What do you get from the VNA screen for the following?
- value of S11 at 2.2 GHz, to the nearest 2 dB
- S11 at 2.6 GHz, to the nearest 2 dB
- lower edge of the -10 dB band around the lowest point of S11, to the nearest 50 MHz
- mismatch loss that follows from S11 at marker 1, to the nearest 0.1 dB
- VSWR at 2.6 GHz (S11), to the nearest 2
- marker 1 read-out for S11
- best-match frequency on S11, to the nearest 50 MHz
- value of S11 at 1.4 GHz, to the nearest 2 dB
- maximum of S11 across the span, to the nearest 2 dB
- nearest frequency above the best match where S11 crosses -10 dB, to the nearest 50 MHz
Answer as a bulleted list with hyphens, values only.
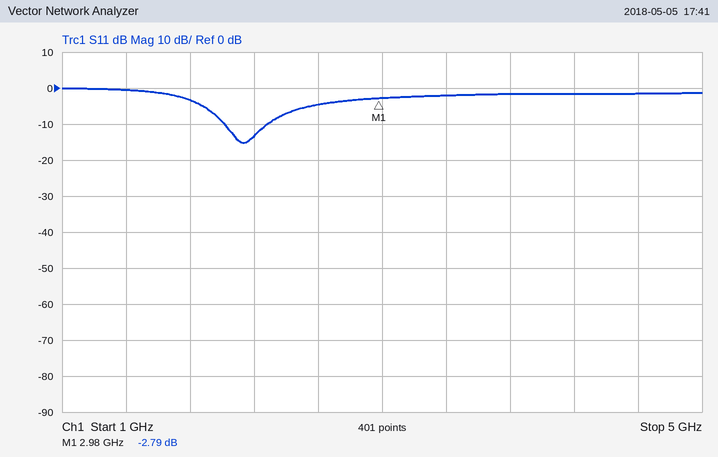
- -14 dB
- -4 dB
- 2.00 GHz
- 3.2 dB
- 4
- -2.79 dB
- 2.15 GHz
- 0 dB
- 0 dB
- 2.30 GHz
